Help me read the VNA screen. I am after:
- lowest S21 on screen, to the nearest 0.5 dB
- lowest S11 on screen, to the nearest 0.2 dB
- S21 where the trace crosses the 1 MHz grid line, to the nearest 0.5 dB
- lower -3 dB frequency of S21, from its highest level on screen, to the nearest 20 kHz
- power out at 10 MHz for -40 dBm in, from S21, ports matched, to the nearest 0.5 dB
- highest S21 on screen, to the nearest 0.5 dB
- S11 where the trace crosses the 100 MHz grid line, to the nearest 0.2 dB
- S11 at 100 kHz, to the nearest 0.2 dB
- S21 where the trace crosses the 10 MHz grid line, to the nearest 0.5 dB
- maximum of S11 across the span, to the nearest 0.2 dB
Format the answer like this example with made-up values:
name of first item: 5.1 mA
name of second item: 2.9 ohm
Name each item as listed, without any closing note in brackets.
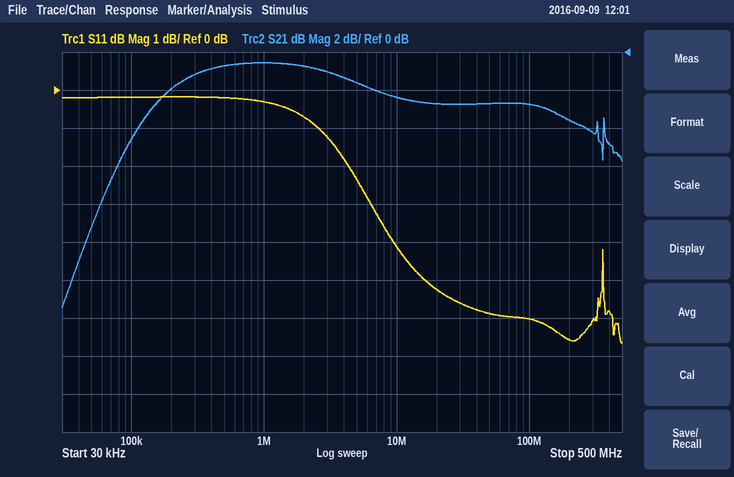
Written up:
lowest S21 on screen, to the nearest 0.5 dB: -13.5 dB
lowest S11 on screen, to the nearest 0.2 dB: -6.6 dB
S21 where the trace crosses the 1 MHz grid line, to the nearest 0.5 dB: -0.5 dB
lower -3 dB frequency of S21, from its highest level on screen, to the nearest 20 kHz: 120 kHz
power out at 10 MHz for -40 dBm in, from S21, ports matched, to the nearest 0.5 dB: -42.5 dBm
highest S21 on screen, to the nearest 0.5 dB: -0.5 dB
S11 where the trace crosses the 100 MHz grid line, to the nearest 0.2 dB: -6.0 dB
S11 at 100 kHz, to the nearest 0.2 dB: -0.2 dB
S21 where the trace crosses the 10 MHz grid line, to the nearest 0.5 dB: -2.5 dB
maximum of S11 across the span, to the nearest 0.2 dB: -0.2 dB
